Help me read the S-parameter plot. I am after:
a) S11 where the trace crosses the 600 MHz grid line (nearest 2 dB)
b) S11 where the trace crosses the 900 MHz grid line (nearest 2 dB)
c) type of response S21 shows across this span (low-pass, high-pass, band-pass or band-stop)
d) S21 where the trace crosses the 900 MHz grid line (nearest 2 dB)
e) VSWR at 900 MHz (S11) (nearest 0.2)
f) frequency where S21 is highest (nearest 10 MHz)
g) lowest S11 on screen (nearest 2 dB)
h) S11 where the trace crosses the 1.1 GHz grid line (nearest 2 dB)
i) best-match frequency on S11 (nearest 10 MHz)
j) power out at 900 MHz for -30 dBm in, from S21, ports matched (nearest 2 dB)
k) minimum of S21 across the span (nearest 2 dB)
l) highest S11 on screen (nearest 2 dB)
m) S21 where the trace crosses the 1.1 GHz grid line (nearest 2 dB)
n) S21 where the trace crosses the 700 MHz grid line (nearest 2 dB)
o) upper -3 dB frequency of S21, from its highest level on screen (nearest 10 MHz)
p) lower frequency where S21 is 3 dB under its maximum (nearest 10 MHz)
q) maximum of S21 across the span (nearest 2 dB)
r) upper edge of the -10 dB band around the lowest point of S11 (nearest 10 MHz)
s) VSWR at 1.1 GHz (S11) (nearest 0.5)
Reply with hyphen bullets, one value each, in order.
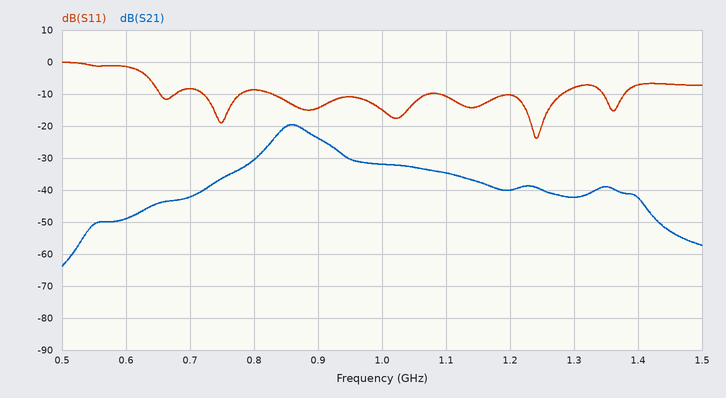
- -2 dB
- -14 dB
- band-pass
- -24 dB
- 1.4
- 860 MHz
- -24 dB
- -10 dB
- 1.24 GHz
- -54 dBm
- -64 dB
- 0 dB
- -34 dB
- -42 dB
- 890 MHz
- 840 MHz
- -20 dB
- 1.28 GHz
- 2.0
